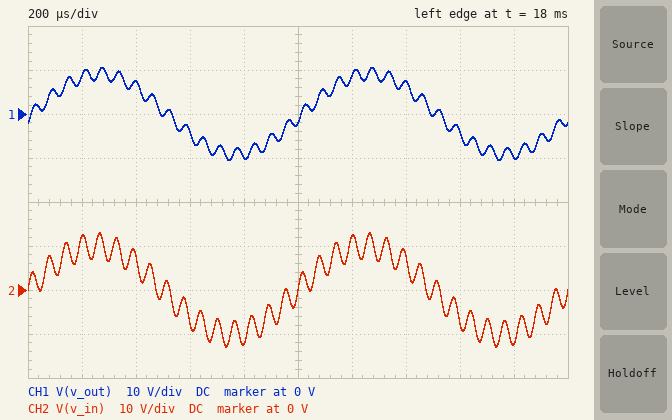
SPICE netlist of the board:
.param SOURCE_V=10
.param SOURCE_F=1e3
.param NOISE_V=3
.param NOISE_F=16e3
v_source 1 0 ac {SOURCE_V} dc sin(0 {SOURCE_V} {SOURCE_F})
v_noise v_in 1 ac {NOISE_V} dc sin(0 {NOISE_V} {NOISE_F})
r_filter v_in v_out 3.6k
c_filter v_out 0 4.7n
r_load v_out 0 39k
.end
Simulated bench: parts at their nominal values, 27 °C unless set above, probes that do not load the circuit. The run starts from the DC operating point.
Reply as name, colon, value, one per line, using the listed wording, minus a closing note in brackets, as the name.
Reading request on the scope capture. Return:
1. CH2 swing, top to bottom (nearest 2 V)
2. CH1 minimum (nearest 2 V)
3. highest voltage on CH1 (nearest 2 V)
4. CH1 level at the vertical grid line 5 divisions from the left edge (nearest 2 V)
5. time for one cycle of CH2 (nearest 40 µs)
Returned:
CH2 swing, top to bottom: 26 V
CH1 minimum: -10 V
highest voltage on CH1: 10 V
CH1 level at the vertical grid line 5 divisions from the left edge: -2 V
time for one cycle of CH2: 1.00 ms
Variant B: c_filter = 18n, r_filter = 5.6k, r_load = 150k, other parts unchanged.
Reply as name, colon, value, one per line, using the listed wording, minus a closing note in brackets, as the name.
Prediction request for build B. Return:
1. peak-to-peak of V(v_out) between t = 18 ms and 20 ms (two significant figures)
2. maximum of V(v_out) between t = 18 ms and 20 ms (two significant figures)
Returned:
peak-to-peak of V(v_out) between t = 18 ms and 20 ms: 17 V
maximum of V(v_out) between t = 18 ms and 20 ms: 8.5 V
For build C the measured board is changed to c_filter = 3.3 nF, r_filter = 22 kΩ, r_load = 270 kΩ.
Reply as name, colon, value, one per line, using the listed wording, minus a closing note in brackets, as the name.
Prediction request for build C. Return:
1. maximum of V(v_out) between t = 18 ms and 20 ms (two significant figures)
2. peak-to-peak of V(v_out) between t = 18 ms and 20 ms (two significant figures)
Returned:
maximum of V(v_out) between t = 18 ms and 20 ms: 8.8 V
peak-to-peak of V(v_out) between t = 18 ms and 20 ms: 18 V
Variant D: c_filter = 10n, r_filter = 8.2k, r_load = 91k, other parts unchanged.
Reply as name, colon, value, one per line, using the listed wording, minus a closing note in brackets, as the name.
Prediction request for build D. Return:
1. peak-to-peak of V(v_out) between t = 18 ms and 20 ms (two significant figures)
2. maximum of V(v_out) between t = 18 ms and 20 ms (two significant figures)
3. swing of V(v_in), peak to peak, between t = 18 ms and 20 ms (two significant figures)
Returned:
peak-to-peak of V(v_out) between t = 18 ms and 20 ms: 17 V
maximum of V(v_out) between t = 18 ms and 20 ms: 8.6 V
swing of V(v_in), peak to peak, between t = 18 ms and 20 ms: 26 V
